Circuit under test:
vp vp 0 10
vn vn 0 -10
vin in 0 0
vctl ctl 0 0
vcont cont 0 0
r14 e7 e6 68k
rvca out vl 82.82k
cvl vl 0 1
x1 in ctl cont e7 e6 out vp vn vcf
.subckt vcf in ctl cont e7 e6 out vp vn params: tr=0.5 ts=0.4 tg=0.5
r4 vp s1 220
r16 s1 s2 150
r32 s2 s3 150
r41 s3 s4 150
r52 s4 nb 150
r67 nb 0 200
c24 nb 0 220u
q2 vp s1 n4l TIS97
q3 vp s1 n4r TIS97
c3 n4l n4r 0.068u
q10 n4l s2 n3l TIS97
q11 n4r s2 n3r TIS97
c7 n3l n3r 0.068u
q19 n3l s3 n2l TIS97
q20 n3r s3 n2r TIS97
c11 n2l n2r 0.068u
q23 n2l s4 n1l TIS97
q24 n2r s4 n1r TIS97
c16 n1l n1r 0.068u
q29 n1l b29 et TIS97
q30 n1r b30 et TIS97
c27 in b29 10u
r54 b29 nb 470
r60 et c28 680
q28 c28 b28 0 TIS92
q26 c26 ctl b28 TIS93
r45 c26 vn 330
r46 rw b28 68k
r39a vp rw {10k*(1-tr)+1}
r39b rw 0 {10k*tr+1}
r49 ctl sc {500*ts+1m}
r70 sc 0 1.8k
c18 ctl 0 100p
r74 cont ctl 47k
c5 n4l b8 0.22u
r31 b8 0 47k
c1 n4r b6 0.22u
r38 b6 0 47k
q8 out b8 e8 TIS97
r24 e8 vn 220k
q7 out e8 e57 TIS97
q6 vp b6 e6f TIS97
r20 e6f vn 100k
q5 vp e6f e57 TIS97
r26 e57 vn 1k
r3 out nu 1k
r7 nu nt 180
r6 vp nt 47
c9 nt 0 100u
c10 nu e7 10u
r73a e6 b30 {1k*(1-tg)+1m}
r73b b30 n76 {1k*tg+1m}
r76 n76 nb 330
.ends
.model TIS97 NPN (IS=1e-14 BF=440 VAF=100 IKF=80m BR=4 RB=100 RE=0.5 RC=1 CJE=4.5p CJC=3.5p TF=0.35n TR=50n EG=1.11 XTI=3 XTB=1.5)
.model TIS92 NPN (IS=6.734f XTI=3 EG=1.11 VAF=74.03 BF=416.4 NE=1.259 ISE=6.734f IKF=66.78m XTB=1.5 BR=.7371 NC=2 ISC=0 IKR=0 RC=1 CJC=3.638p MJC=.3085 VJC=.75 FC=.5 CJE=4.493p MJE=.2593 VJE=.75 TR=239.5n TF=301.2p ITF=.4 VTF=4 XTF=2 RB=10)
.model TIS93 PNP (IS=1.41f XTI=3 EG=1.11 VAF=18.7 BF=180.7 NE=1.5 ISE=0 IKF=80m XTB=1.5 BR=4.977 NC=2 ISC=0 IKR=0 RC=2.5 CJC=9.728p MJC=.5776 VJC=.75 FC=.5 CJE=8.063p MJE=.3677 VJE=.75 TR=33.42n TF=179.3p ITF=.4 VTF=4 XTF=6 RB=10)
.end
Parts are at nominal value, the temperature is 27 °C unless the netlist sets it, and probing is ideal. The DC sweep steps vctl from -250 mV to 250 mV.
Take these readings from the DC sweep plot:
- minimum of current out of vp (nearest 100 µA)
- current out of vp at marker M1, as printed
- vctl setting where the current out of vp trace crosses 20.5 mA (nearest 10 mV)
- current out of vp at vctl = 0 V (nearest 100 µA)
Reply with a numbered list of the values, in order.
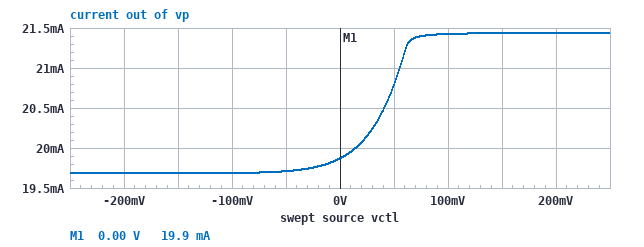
1. 19.7 mA
2. 19.9 mA
3. 40 mV
4. 19.9 mA
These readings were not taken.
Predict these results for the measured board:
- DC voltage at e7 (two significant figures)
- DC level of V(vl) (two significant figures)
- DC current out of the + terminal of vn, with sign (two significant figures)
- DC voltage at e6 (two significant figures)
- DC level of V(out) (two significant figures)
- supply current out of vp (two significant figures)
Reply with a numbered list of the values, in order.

1. 2.0 V
2. 3.2 V
3. -8.9 mA
4. 2.0 V
5. 3.2 V
6. 20 mA
